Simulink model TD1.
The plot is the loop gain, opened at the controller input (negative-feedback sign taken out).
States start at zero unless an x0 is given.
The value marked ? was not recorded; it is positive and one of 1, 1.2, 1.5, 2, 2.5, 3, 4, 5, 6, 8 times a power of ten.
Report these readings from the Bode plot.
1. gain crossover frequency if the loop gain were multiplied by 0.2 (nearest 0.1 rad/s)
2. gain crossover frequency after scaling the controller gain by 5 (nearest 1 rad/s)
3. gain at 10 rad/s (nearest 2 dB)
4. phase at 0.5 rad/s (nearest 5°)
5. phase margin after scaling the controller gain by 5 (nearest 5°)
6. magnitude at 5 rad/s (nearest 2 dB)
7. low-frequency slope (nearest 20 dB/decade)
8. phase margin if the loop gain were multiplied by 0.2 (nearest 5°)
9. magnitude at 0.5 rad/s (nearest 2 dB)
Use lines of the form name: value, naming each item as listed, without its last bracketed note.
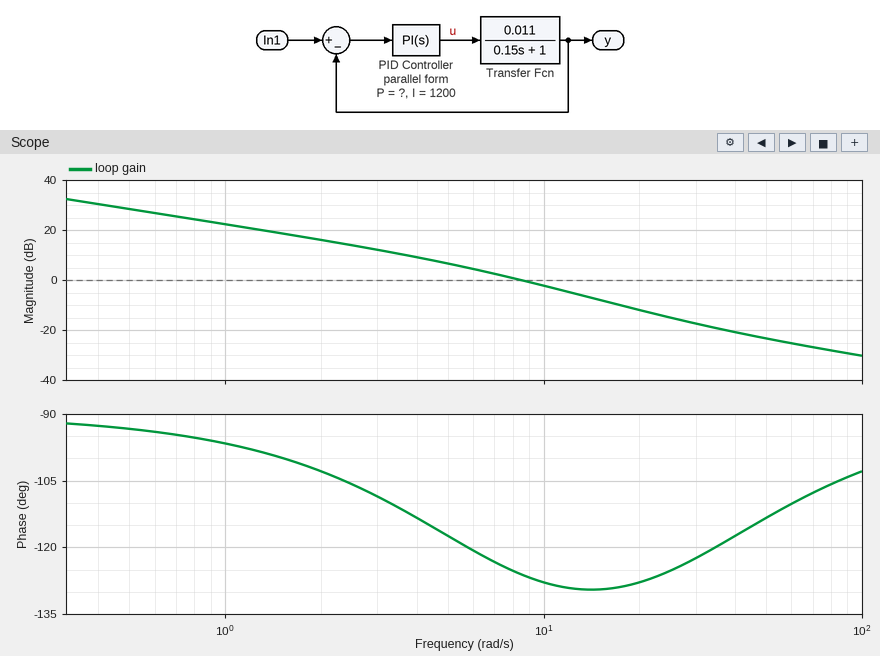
gain crossover frequency if the loop gain were multiplied by 0.2: 2.5 rad/s
gain crossover frequency after scaling the controller gain by 5: 23 rad/s
gain at 10 rad/s: -2 dB
phase at 0.5 rad/s: -95°
phase margin after scaling the controller gain by 5: 55°
magnitude at 5 rad/s: 6 dB
low-frequency slope: -20 dB/decade
phase margin if the loop gain were multiplied by 0.2: 75°
magnitude at 0.5 rad/s: 28 dB
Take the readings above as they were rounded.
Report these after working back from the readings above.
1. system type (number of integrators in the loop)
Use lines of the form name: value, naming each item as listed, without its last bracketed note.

system type: 1
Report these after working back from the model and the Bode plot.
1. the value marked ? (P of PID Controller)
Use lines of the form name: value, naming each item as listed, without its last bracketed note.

the value marked ?: 40
